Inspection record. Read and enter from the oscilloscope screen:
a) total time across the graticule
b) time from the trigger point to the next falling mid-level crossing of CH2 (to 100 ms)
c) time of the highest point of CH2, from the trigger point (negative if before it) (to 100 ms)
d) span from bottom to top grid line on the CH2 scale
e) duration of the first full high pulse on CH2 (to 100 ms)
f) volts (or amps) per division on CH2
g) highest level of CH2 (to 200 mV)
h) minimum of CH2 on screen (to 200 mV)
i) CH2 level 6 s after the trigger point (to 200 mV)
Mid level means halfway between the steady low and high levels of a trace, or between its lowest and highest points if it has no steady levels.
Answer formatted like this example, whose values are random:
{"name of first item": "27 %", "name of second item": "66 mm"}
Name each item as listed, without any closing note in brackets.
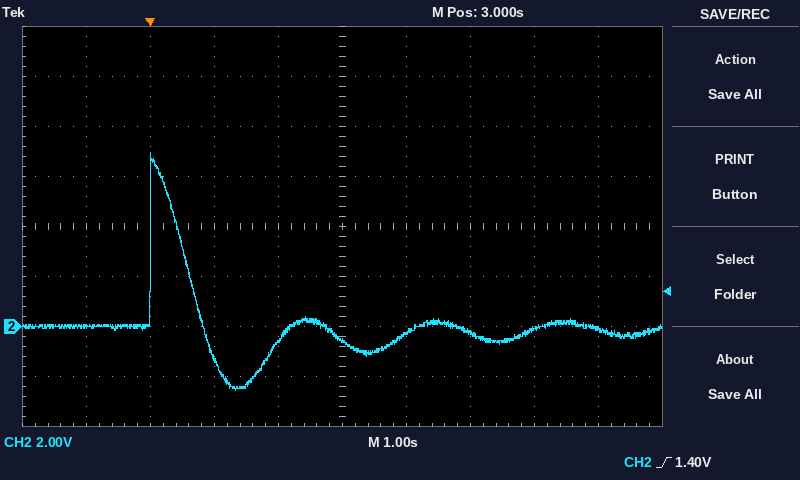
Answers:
{"total time across the graticule": "10 s", "time from the trigger point to the next falling mid-level crossing of CH2": "600 ms", "time of the highest point of CH2, from the trigger point (negative if before it)": "0.0 s", "span from bottom to top grid line on the CH2 scale": "16 V", "duration of the first full high pulse on CH2": "600 ms", "volts (or amps) per division on CH2": "2 V", "highest level of CH2": "7.0 V", "minimum of CH2 on screen": "-2.6 V", "CH2 level 6 s after the trigger point": "-200 mV"}
